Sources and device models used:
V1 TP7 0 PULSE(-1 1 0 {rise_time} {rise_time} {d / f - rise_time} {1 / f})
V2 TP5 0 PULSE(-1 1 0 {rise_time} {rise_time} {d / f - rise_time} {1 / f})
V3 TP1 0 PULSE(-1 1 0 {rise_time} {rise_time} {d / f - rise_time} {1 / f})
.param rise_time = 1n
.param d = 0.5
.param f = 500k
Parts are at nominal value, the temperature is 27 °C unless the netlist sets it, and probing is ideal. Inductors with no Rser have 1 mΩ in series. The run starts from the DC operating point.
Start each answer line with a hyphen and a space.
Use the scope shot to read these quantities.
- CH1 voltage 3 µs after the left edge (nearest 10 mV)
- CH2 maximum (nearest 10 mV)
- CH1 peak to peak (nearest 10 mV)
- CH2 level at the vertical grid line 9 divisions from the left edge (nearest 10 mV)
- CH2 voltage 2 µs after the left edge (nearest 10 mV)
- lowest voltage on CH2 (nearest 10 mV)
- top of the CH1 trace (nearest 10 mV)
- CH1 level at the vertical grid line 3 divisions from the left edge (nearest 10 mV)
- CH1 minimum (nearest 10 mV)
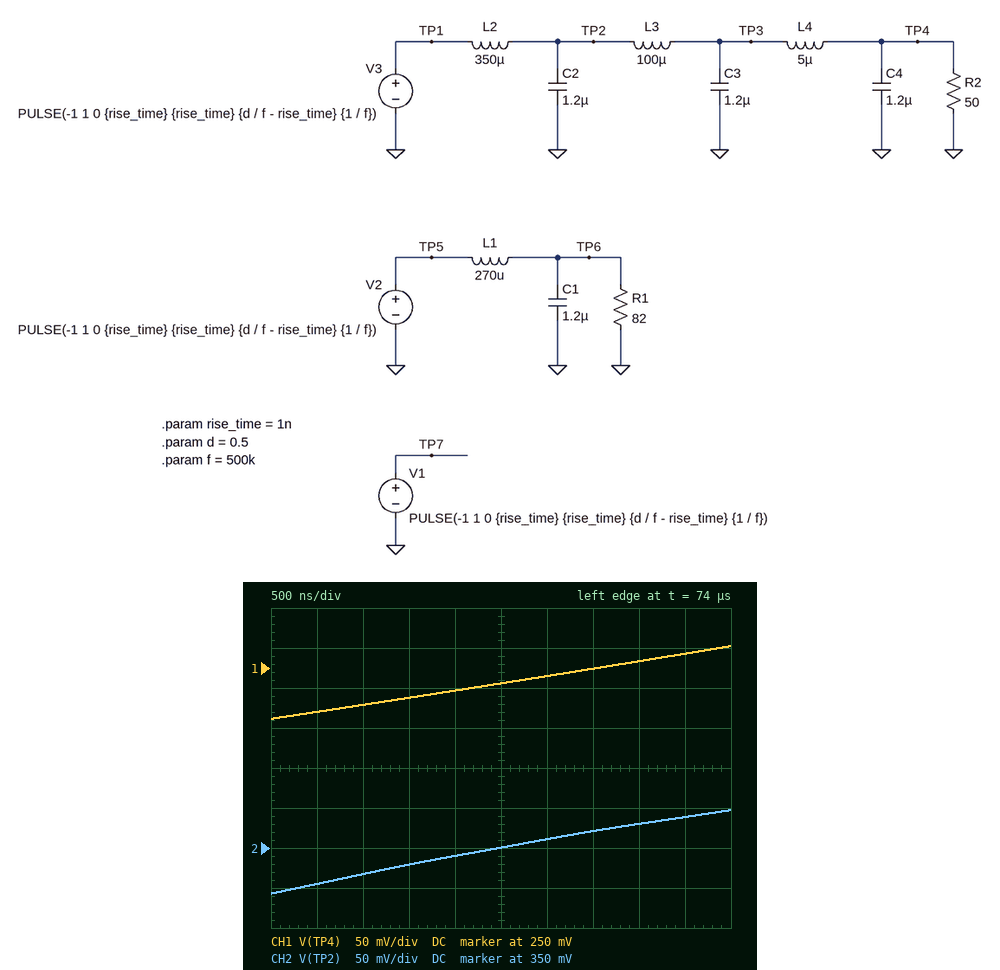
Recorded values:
- 240 mV
- 400 mV
- 90 mV
- 390 mV
- 340 mV
- 290 mV
- 280 mV
- 210 mV
- 190 mV
